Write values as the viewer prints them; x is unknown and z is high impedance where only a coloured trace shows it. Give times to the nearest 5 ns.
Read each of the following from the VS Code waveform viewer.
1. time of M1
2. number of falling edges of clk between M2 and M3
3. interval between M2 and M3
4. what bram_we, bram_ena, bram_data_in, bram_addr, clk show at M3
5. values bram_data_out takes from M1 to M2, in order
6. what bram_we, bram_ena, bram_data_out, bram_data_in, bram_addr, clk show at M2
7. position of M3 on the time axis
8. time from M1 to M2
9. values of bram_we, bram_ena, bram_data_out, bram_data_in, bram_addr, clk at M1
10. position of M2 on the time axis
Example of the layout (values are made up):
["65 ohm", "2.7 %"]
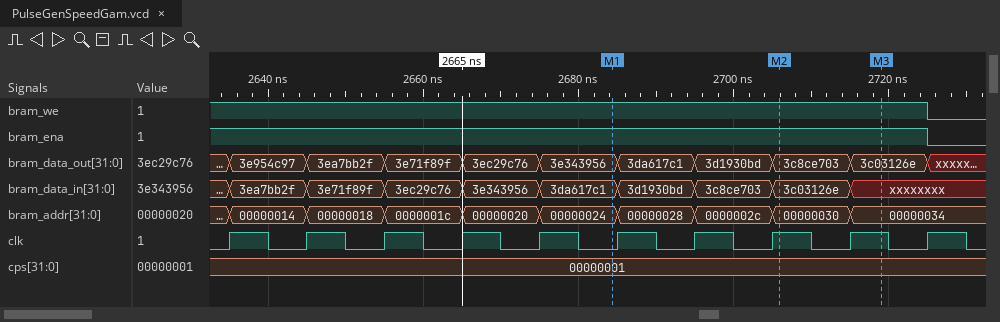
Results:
["2685 ns", "1", "15 ns", "bram_we=1, bram_ena=1, bram_data_in=xxxxxxxx, bram_addr=00000034, clk=1", "3e343956, 3da617c1, 3d1930bd, 3c8ce703", "bram_we=1, bram_ena=1, bram_data_out=3c8ce703, bram_data_in=3c03126e, bram_addr=00000030, clk=1", "2720 ns", "20 ns", "bram_we=1, bram_ena=1, bram_data_out=3e343956, bram_data_in=3da617c1, bram_addr=00000024, clk=0", "2705 ns"]
